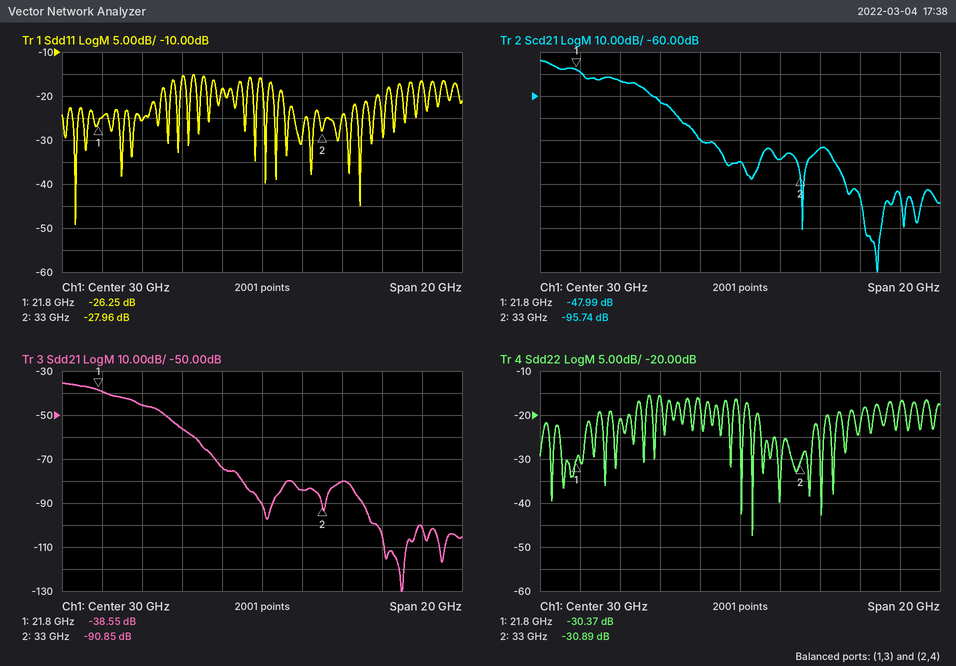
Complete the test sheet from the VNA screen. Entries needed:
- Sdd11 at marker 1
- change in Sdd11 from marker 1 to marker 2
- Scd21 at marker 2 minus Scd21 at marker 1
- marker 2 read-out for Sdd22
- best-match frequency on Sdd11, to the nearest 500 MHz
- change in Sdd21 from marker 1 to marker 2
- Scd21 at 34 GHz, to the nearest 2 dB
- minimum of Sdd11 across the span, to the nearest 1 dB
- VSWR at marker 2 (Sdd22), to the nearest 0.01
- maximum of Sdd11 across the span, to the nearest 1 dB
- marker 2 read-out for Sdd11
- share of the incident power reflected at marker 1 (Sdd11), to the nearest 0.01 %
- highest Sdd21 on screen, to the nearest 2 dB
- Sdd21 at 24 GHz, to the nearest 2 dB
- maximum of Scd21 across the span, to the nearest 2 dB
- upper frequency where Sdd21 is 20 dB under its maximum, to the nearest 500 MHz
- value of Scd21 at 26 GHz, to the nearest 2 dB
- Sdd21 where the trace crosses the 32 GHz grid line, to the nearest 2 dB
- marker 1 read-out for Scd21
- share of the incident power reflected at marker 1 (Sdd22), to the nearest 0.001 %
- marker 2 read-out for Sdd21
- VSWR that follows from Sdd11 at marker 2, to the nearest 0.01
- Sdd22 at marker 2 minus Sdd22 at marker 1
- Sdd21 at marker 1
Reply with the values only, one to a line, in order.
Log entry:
-26.25 dB
-1.71 dB
-47.75 dB
-30.89 dB
20.5 GHz
-52.30 dB
-84 dB
-49 dB
1.06
-15 dB
-27.96 dB
0.24 %
-36 dB
-46 dB
-44 dB
26.0 GHz
-62 dB
-84 dB
-47.99 dB
0.092 %
-90.85 dB
1.08
-0.52 dB
-38.55 dB
